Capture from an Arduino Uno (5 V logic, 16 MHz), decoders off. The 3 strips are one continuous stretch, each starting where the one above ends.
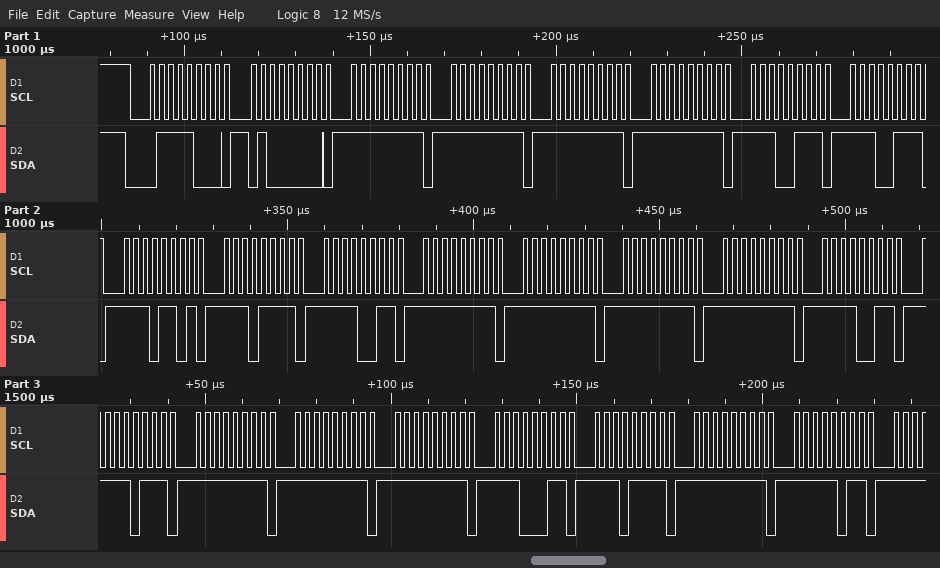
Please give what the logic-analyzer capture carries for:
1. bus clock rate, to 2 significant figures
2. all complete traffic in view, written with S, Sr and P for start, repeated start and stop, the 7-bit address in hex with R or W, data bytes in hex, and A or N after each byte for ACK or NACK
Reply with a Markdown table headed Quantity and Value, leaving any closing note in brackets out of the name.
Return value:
| Quantity | Value |
|---|---|
| bus clock rate, to 2 significant figures | 400 kHz |
| all complete traffic in view, written with S, Sr and P for start, repeated start and stop, the 7-bit address in hex with R or W, data bytes in hex, and A or N after each byte for ACK or NACK | S 3CW A 40 A FF A FF A FF A FF A E7 A E7 A ED A EF A F3 A FF A FF A FF A FF A F3 A F7 A FF A FF A FF A E3 A EF A FF A FB A |
